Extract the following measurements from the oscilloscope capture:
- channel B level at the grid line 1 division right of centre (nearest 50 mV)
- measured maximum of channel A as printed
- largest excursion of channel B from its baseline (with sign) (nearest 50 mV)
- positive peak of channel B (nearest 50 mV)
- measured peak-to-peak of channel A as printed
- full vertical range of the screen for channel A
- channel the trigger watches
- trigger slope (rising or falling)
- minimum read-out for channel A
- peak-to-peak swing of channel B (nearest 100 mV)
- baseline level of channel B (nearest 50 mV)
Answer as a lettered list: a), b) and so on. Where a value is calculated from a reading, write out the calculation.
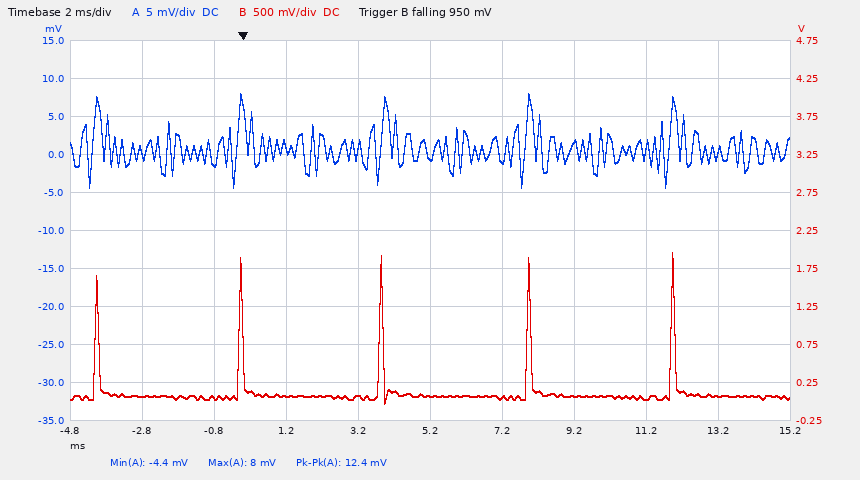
a) 50 mV
b) 8 mV
c) 1.95 V − (50 mV) = +1.90 V
d) 1.95 V
e) 12.4 mV
f) 50 mV
g) channel B
h) falling
i) -4.4 mV
j) 2.00 V
k) 50 mV
